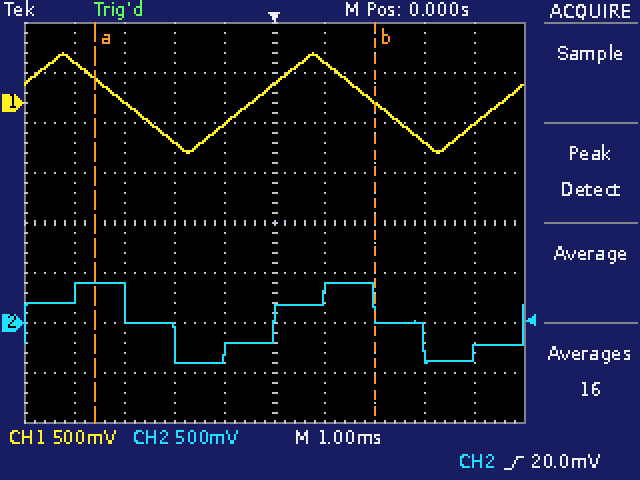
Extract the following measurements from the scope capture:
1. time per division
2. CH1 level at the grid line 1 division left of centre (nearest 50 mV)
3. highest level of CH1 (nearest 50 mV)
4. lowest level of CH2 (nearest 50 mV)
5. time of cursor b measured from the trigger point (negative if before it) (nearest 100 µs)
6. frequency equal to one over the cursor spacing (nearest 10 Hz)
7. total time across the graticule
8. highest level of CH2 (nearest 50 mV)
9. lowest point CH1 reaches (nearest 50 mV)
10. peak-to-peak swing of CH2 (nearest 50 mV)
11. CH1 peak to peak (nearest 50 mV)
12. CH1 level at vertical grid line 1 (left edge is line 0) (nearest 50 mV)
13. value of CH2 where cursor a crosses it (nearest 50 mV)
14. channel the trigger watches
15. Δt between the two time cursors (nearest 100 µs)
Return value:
1 ms
-200 mV
500 mV
-400 mV
+2.0 ms
180 Hz
10 ms
400 mV
-500 mV
800 mV
1.00 V
400 mV
400 mV
CH2
5.6 ms
